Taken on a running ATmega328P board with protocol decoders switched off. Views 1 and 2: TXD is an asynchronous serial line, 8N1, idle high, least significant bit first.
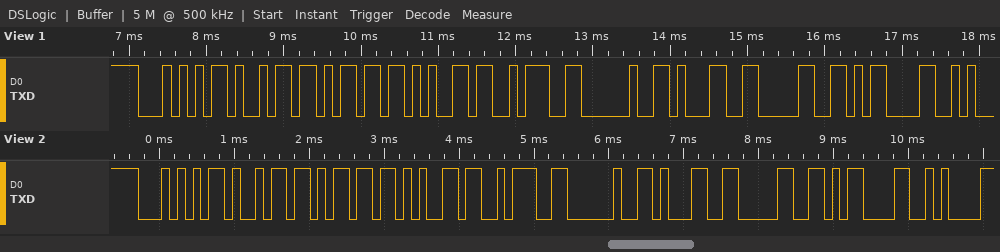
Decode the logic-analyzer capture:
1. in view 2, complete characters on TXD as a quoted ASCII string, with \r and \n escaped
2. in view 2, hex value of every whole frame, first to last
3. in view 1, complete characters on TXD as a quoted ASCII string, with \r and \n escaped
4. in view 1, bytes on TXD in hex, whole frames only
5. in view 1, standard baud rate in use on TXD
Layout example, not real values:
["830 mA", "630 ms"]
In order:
["\"Time: 10\\r\\n\"", "54 69 6D 65 3A 20 31 30 0D 0A", "\"Time: 10\\r\"", "0x54 0x69 0x6D 0x65 0x3A 0x20 0x31 0x30 0x0D", "9600 baud"]
